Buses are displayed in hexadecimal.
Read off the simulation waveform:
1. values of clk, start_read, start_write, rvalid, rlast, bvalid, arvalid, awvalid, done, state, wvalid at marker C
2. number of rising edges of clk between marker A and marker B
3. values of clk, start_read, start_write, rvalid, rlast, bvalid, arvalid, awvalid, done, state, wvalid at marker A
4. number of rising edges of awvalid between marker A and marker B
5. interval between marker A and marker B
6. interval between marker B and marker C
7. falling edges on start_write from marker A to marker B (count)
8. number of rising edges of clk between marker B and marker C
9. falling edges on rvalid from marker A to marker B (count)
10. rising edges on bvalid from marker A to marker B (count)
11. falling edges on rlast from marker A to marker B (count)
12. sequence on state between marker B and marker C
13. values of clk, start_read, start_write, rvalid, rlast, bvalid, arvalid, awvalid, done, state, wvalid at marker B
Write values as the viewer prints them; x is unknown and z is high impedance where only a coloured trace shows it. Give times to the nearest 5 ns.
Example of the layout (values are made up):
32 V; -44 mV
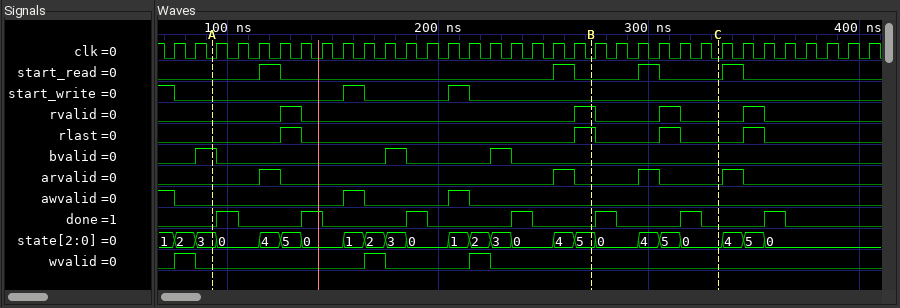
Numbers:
clk=0, start_read=0, start_write=0, rvalid=0, rlast=0, bvalid=0, arvalid=0, awvalid=0, done=0, state=0, wvalid=0; 18; clk=0, start_read=0, start_write=0, rvalid=0, rlast=0, bvalid=1, arvalid=0, awvalid=0, done=0, state=3, wvalid=0; 2; 180 ns; 60 ns; 2; 6; 1; 2; 1; 5, 0, 4, 5, 0; clk=0, start_read=0, start_write=0, rvalid=1, rlast=1, bvalid=0, arvalid=0, awvalid=0, done=0, state=5, wvalid=0
